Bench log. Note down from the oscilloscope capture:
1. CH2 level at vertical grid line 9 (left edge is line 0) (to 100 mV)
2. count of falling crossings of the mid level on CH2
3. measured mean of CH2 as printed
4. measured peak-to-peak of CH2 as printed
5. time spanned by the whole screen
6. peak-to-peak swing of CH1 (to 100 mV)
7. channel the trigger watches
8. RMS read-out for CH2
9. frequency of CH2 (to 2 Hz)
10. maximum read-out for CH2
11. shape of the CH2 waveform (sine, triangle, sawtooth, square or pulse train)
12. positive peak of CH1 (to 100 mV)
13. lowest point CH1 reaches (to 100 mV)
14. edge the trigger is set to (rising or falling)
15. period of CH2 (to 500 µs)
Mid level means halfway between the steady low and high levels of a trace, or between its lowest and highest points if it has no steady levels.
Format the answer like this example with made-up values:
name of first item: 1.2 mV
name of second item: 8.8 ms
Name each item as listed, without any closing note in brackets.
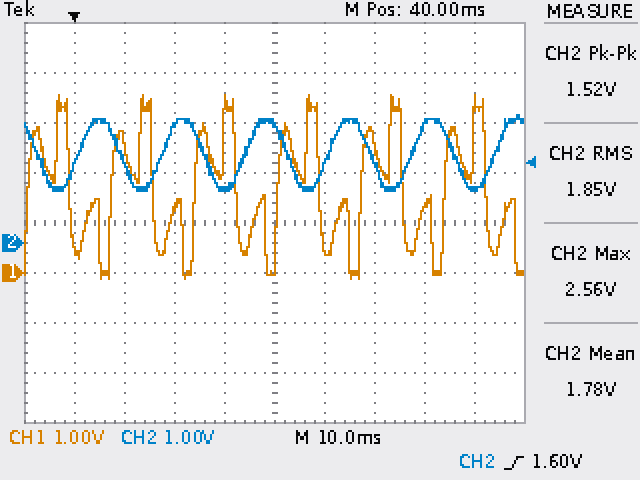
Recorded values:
CH2 level at vertical grid line 9 (left edge is line 0): 1.1 V
count of falling crossings of the mid level on CH2: 6
measured mean of CH2 as printed: 1.78 V
measured peak-to-peak of CH2 as printed: 1.52 V
time spanned by the whole screen: 100 ms
peak-to-peak swing of CH1: 3.7 V
channel the trigger watches: CH2
RMS read-out for CH2: 1.85 V
frequency of CH2: 60 Hz
maximum read-out for CH2: 2.56 V
shape of the CH2 waveform: sine
positive peak of CH1: 3.6 V
lowest point CH1 reaches: -100 mV
edge the trigger is set to: rising
period of CH2: 16.5 ms
